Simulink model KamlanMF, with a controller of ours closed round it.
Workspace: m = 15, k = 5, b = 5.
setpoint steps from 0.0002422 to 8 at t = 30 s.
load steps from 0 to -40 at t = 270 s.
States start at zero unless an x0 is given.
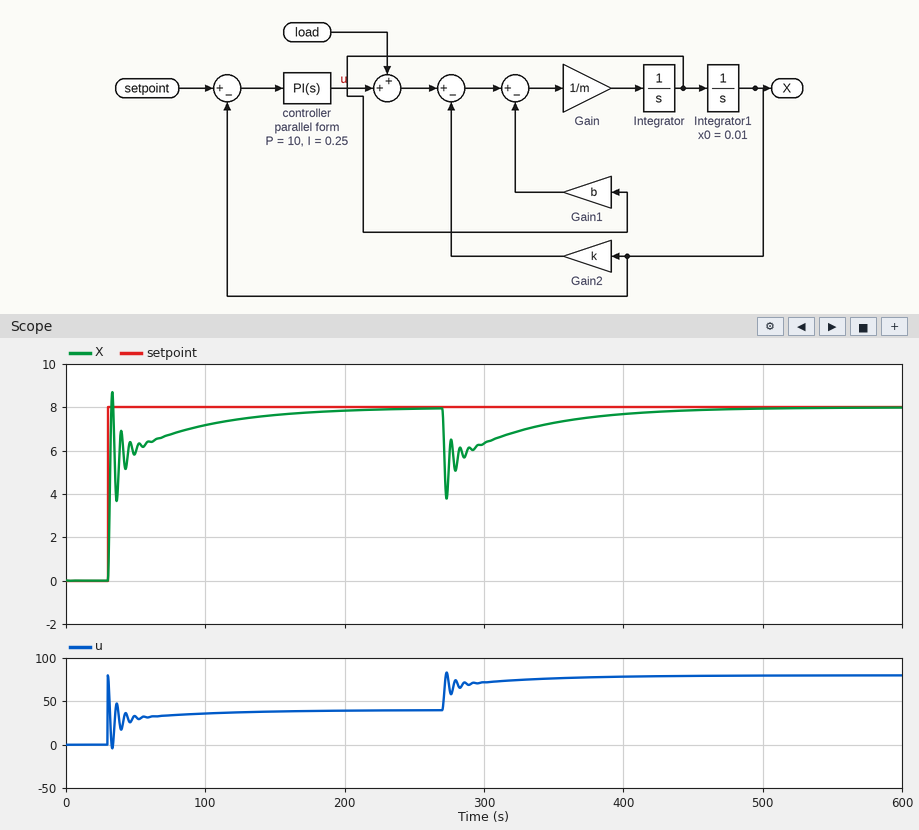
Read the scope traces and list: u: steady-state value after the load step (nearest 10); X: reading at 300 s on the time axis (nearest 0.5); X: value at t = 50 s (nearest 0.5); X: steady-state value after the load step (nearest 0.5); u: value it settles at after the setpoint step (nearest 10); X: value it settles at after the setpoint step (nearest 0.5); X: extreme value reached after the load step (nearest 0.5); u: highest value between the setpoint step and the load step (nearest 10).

80
6.5
6.0
8.0
40
8.0
4.0
80
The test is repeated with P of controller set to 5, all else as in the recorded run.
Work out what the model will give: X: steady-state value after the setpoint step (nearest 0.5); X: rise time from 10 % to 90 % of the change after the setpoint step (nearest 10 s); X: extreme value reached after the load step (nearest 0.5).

8.0
60 s
2.0
